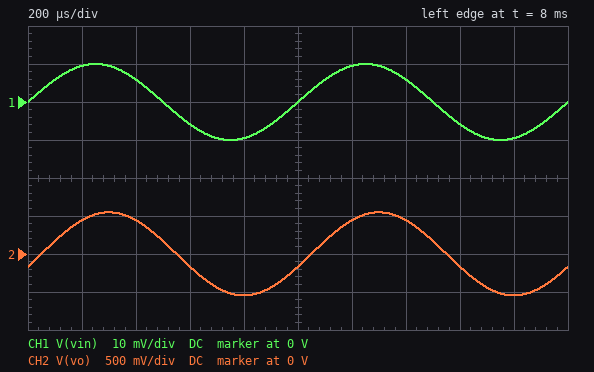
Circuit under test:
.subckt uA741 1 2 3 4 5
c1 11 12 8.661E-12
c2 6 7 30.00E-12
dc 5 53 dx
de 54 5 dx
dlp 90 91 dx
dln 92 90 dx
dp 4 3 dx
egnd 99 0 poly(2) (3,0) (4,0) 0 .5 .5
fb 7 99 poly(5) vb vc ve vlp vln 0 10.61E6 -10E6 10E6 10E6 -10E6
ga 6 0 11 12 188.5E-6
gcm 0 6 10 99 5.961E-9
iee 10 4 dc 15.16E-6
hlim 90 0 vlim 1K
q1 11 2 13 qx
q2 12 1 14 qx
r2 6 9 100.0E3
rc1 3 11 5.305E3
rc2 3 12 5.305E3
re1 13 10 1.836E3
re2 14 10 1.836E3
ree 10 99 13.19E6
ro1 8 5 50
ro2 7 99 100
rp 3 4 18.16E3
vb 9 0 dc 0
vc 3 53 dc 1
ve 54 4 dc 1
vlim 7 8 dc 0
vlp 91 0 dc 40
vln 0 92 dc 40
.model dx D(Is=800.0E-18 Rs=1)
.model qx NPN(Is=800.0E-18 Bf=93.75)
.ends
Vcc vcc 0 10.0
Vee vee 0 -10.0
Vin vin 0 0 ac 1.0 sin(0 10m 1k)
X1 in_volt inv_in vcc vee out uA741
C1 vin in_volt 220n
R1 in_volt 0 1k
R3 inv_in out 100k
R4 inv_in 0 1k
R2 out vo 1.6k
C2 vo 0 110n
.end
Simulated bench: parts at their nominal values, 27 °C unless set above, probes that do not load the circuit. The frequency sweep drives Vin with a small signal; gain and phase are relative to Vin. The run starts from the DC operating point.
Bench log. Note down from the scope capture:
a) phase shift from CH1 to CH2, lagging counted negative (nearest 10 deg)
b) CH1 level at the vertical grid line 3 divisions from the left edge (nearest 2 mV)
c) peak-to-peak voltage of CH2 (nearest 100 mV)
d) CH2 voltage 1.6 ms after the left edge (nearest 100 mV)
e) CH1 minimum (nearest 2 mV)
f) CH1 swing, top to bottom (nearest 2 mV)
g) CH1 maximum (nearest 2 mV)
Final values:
-20 deg
-6 mV
1.1 V
-200 mV
-10 mV
20 mV
10 mV
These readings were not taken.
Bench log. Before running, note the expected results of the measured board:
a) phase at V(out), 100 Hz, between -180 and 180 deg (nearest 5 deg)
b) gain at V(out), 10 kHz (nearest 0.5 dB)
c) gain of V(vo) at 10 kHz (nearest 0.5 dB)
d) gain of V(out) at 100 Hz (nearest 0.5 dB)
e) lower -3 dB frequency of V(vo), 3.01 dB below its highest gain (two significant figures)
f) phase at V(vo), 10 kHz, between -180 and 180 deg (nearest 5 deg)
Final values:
80 deg
37.0 dB
16.0 dB
23.0 dB
330 Hz
-125 deg
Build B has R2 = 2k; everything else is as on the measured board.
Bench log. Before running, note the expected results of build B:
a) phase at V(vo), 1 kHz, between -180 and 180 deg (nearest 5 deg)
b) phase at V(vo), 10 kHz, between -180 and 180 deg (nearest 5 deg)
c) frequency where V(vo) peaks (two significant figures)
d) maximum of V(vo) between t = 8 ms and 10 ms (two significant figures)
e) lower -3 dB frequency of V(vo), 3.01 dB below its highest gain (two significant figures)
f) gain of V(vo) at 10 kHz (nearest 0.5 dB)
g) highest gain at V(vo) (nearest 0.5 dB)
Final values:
-25 deg
-130 deg
720 Hz
480 mV
300 Hz
14.0 dB
34.0 dB
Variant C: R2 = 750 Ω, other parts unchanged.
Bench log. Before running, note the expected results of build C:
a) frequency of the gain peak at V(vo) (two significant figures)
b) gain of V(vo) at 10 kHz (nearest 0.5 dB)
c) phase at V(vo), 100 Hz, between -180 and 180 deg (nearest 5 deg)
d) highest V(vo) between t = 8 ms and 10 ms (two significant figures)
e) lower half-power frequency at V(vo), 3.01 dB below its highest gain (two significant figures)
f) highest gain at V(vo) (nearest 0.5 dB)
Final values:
1.2 kHz
22.5 dB
80 deg
730 mV
450 Hz
37.5 dB
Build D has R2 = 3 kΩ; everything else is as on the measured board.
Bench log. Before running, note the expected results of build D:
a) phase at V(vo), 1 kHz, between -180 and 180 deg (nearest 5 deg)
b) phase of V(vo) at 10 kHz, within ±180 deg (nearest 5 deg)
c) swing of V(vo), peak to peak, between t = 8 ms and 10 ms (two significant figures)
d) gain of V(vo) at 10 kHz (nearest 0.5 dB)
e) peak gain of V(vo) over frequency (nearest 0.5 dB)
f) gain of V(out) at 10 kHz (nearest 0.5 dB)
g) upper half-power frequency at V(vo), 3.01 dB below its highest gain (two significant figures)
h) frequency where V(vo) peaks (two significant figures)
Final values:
-35 deg
-130 deg
710 mV
10.5 dB
32.0 dB
37.0 dB
1.4 kHz
590 Hz
